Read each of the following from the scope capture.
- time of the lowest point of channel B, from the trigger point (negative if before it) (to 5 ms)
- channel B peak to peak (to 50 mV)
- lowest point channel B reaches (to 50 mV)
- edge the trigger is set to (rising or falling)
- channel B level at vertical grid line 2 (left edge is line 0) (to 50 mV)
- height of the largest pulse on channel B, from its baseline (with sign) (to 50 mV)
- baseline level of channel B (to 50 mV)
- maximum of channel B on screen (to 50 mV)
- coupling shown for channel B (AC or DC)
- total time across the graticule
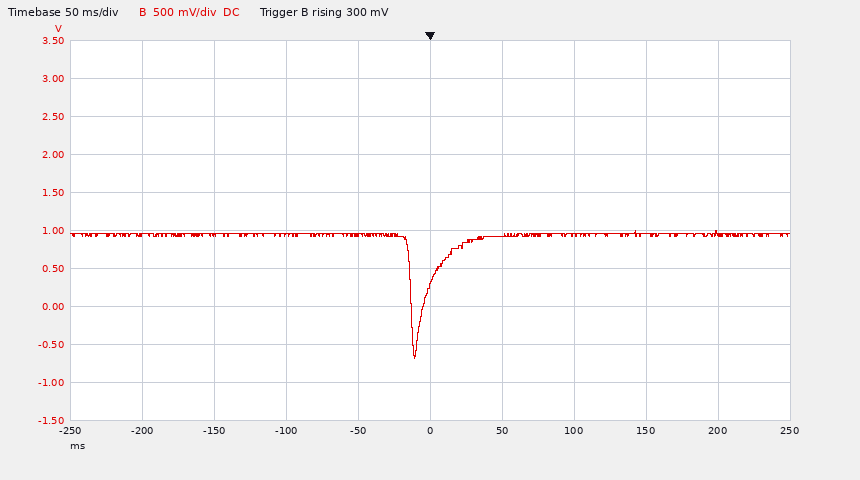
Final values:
-10 ms
1.70 V
-700 mV
rising
950 mV
-1.65 V
950 mV
1.00 V
DC
500 ms
